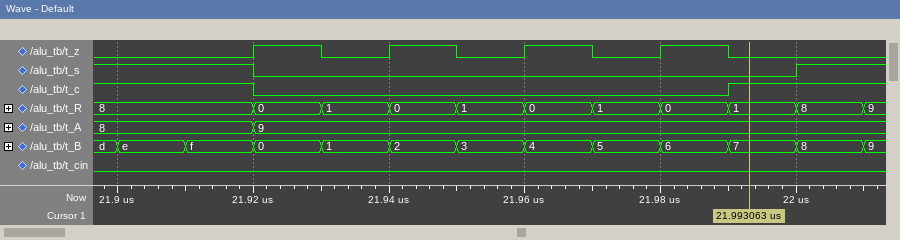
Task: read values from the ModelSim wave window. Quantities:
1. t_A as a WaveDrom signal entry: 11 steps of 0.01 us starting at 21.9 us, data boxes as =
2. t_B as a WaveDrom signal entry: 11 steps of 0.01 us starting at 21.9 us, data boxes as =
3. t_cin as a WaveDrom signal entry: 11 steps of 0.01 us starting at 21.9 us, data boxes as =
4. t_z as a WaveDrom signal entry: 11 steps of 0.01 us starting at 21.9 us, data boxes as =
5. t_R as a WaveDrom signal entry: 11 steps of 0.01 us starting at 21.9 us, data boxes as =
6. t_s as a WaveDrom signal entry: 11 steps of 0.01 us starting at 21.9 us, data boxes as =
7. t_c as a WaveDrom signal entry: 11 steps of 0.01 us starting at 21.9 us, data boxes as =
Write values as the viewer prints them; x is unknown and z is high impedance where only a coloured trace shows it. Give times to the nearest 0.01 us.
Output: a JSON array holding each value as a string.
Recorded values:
["{name: 't_A', wave: '=.=........', data: '8 9'}", "{name: 't_B', wave: '===========', data: 'e f 0 1 2 3 4 5 6 7 8'}", "{name: 't_cin', wave: '0..........'}", "{name: 't_z', wave: '0.10101010.'}", "{name: 't_R', wave: '=.=========', data: '8 0 1 0 1 0 1 0 1 8'}", "{name: 't_s', wave: '1.0.......1'}", "{name: 't_c', wave: '1.0......1.'}"]
